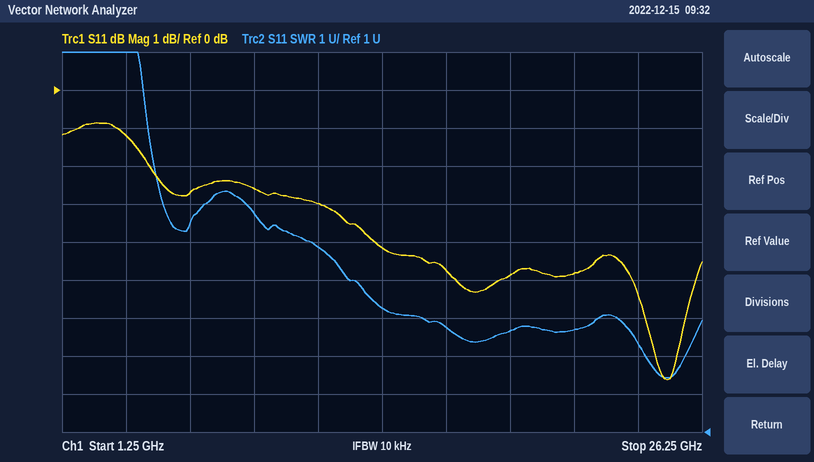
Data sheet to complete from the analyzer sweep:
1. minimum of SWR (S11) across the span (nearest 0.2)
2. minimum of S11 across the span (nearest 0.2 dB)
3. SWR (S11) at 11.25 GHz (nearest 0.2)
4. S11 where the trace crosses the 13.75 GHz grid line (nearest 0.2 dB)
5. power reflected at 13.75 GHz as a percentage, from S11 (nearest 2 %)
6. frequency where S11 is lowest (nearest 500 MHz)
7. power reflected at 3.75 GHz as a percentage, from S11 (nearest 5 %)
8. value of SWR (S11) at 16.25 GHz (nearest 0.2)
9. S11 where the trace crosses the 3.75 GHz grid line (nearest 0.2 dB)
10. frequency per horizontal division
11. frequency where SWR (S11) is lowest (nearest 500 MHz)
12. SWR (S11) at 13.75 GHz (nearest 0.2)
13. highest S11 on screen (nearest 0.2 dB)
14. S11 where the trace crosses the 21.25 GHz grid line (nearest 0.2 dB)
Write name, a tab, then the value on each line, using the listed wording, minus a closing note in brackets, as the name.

minimum of SWR (S11) across the span	2.4
minimum of S11 across the span	-7.6 dB
SWR (S11) at 11.25 GHz	5.8
S11 where the trace crosses the 13.75 GHz grid line	-4.2 dB
power reflected at 13.75 GHz as a percentage, from S11	38 %
frequency where S11 is lowest	25.0 GHz
power reflected at 3.75 GHz as a percentage, from S11	75 %
value of SWR (S11) at 16.25 GHz	3.8
S11 where the trace crosses the 3.75 GHz grid line	-1.2 dB
frequency per horizontal division	2.5 GHz
frequency where SWR (S11) is lowest	25.0 GHz
SWR (S11) at 13.75 GHz	4.2
highest S11 on screen	-0.8 dB
S11 where the trace crosses the 21.25 GHz grid line	-4.8 dB
